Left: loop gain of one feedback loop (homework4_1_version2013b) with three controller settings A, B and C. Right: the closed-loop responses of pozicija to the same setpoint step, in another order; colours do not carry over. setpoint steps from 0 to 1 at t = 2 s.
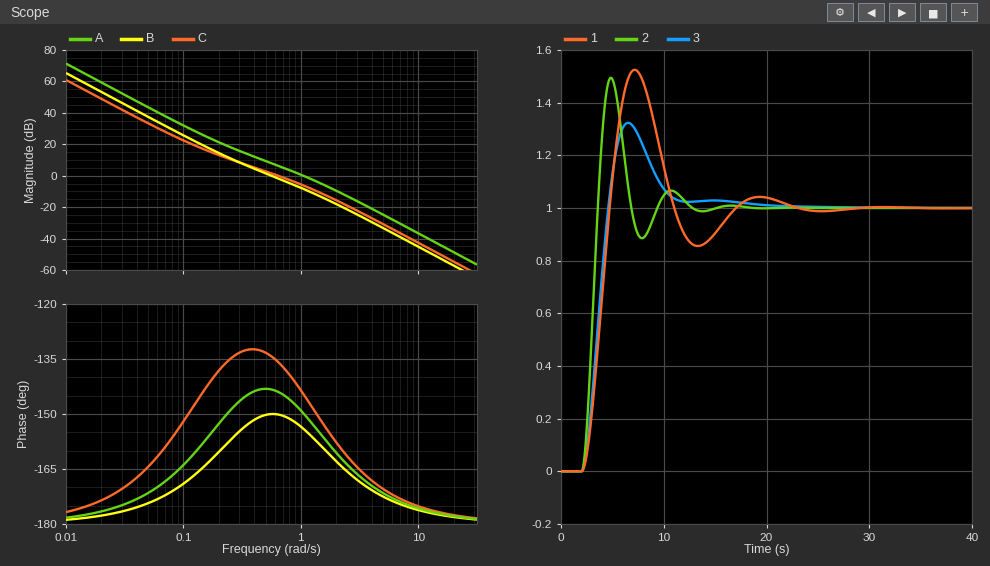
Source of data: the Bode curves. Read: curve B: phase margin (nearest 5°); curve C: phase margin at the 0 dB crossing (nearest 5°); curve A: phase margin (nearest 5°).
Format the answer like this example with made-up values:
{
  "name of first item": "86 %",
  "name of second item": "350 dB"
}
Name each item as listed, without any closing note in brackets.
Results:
{
  "curve B: phase margin": "30°",
  "curve C: phase margin at the 0 dB crossing": "45°",
  "curve A: phase margin": "30°"
}
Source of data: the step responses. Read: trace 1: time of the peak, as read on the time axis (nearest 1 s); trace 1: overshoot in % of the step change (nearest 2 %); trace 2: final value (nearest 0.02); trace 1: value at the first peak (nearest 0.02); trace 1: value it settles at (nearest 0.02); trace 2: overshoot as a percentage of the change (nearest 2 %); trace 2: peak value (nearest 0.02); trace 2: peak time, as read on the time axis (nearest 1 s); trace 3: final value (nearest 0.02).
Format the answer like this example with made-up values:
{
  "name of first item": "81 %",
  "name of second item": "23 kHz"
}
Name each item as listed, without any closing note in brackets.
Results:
{
  "trace 1: time of the peak, as read on the time axis": "7 s",
  "trace 1: overshoot in % of the step change": "52 %",
  "trace 2: final value": "1.00",
  "trace 1: value at the first peak": "1.52",
  "trace 1: value it settles at": "1.00",
  "trace 2: overshoot as a percentage of the change": "50 %",
  "trace 2: peak value": "1.50",
  "trace 2: peak time, as read on the time axis": "5 s",
  "trace 3: final value": "1.00"
}
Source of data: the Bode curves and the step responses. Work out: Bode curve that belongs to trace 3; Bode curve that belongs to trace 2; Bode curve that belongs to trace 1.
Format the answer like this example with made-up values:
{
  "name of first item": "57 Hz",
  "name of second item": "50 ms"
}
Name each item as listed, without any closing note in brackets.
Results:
{
  "Bode curve that belongs to trace 3": "C",
  "Bode curve that belongs to trace 2": "A",
  "Bode curve that belongs to trace 1": "B"
}
